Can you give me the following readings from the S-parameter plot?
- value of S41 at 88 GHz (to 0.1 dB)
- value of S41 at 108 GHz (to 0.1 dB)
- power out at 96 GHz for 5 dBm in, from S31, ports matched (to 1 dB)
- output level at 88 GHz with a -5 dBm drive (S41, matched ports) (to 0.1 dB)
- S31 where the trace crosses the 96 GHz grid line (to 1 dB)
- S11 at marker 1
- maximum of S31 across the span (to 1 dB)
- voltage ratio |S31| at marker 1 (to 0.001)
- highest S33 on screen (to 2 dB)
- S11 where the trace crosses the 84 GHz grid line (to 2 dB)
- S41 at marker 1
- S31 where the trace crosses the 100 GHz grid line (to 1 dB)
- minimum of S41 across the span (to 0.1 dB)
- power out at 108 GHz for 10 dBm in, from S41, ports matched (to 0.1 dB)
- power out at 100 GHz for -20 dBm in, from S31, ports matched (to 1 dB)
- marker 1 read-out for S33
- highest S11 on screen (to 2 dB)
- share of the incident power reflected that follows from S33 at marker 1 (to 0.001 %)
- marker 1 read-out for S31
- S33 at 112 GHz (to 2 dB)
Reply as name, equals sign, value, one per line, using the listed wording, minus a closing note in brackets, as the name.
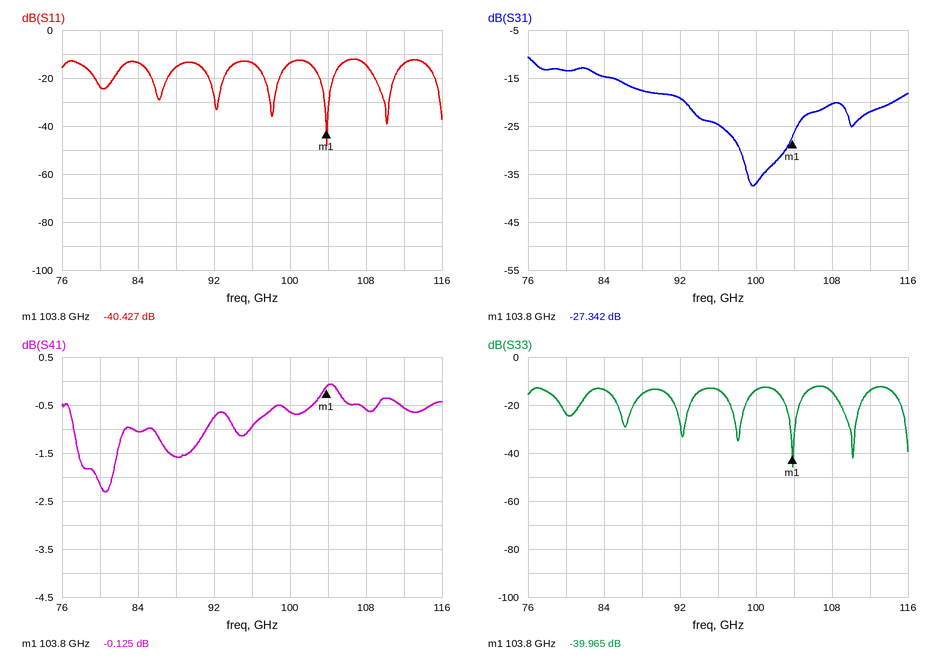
value of S41 at 88 GHz = -1.6 dB
value of S41 at 108 GHz = -0.6 dB
power out at 96 GHz for 5 dBm in, from S31, ports matched = -20 dBm
output level at 88 GHz with a -5 dBm drive (S41, matched ports) = -6.6 dBm
S31 where the trace crosses the 96 GHz grid line = -25 dB
S11 at marker 1 = -40.427 dB
maximum of S31 across the span = -11 dB
voltage ratio |S31| at marker 1 = 0.043
highest S33 on screen = -12 dB
S11 where the trace crosses the 84 GHz grid line = -14 dB
S41 at marker 1 = -0.125 dB
S31 where the trace crosses the 100 GHz grid line = -37 dB
minimum of S41 across the span = -2.3 dB
power out at 108 GHz for 10 dBm in, from S41, ports matched = 9.4 dBm
power out at 100 GHz for -20 dBm in, from S31, ports matched = -57 dBm
marker 1 read-out for S33 = -39.965 dB
highest S11 on screen = -12 dB
share of the incident power reflected that follows from S33 at marker 1 = 0.010 %
marker 1 read-out for S31 = -27.342 dB
S33 at 112 GHz = -14 dB
